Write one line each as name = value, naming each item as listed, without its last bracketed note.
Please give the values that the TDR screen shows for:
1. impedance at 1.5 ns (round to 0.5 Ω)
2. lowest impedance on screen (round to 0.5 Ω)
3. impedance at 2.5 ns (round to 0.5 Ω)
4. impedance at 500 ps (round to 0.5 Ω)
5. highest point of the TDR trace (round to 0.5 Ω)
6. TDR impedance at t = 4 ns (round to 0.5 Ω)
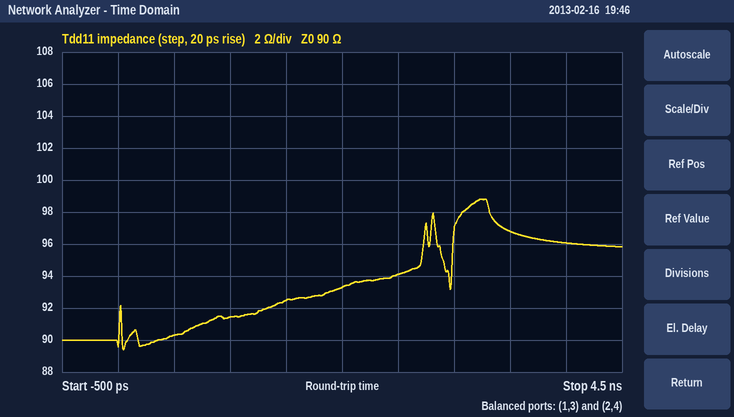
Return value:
impedance at 1.5 ns = 92.5 Ω
lowest impedance on screen = 89.5 Ω
impedance at 2.5 ns = 94.0 Ω
impedance at 500 ps = 90.5 Ω
highest point of the TDR trace = 99.0 Ω
TDR impedance at t = 4 ns = 96.0 Ω
